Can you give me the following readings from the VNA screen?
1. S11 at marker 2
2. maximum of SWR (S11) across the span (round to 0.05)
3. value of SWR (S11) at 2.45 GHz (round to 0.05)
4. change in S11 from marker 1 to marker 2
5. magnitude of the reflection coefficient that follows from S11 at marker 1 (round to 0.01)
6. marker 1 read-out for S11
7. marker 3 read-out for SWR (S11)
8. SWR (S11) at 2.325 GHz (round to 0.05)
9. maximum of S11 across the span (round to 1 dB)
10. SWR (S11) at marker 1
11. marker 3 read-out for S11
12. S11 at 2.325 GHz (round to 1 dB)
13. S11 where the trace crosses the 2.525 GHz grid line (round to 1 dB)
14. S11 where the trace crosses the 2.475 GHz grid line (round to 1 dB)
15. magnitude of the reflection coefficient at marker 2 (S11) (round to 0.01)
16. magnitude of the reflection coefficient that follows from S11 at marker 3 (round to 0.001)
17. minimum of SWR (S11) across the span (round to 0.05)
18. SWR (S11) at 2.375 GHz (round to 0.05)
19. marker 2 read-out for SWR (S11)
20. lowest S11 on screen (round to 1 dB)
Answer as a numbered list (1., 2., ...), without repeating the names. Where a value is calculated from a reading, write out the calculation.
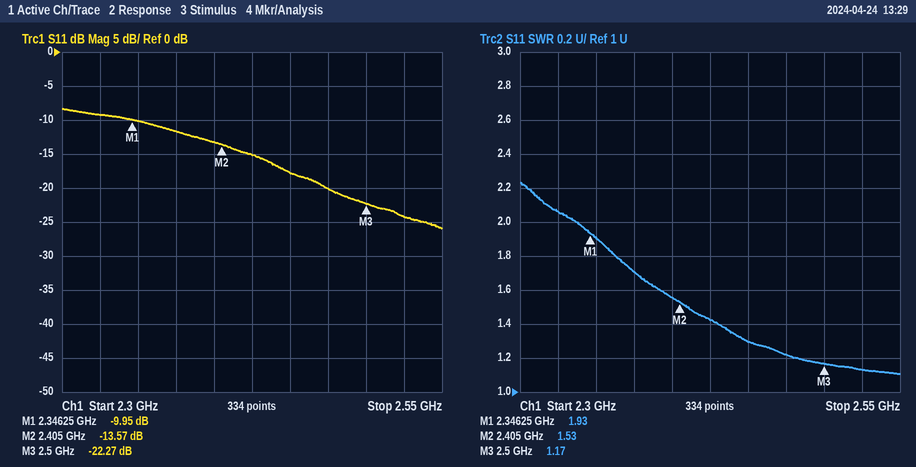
1. -13.57 dB
2. 2.25
3. 1.30
4. -13.57 − (-9.95) = -3.62 dB
5. 10^(-9.95/20) ≈ 0.32
6. -9.95 dB
7. 1.17
8. 2.05
9. -8 dB
10. 1.93
11. -22.27 dB
12. -9 dB
13. -24 dB
14. -20 dB
15. 10^(-13.57/20) ≈ 0.21
16. 10^(-22.27/20) ≈ 0.077
17. 1.10
18. 1.70
19. 1.53
20. -26 dB
